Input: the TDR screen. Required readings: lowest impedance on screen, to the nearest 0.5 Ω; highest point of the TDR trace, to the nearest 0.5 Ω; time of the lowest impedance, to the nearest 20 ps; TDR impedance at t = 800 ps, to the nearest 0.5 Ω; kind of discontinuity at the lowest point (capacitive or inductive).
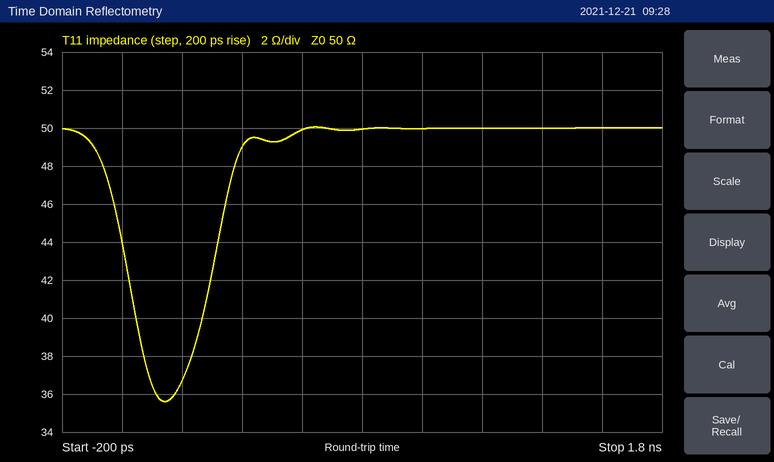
35.5 Ω
50.0 Ω
140 ps
50.0 Ω
capacitive
